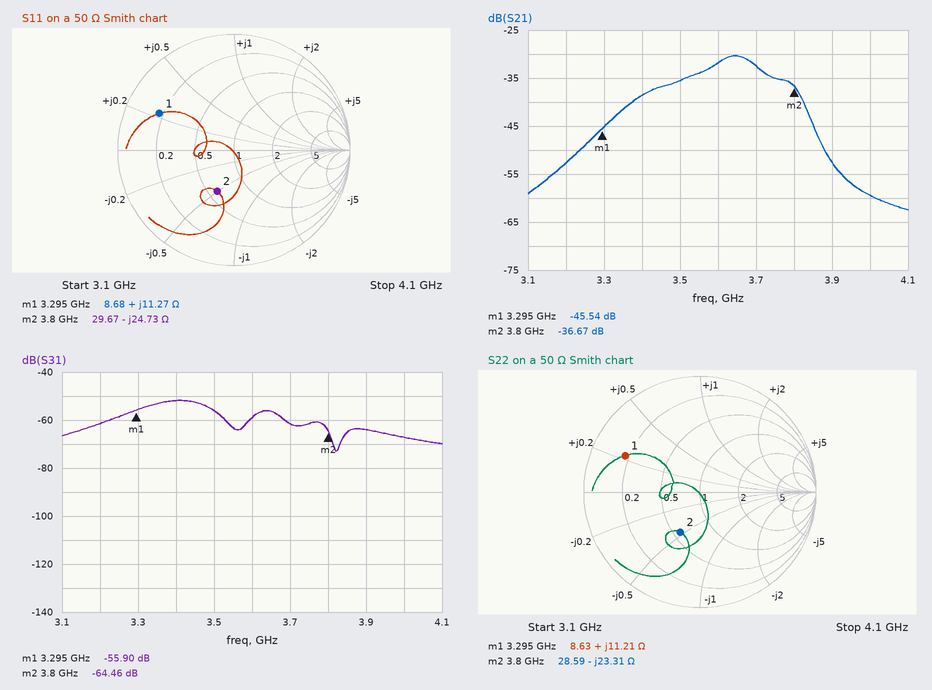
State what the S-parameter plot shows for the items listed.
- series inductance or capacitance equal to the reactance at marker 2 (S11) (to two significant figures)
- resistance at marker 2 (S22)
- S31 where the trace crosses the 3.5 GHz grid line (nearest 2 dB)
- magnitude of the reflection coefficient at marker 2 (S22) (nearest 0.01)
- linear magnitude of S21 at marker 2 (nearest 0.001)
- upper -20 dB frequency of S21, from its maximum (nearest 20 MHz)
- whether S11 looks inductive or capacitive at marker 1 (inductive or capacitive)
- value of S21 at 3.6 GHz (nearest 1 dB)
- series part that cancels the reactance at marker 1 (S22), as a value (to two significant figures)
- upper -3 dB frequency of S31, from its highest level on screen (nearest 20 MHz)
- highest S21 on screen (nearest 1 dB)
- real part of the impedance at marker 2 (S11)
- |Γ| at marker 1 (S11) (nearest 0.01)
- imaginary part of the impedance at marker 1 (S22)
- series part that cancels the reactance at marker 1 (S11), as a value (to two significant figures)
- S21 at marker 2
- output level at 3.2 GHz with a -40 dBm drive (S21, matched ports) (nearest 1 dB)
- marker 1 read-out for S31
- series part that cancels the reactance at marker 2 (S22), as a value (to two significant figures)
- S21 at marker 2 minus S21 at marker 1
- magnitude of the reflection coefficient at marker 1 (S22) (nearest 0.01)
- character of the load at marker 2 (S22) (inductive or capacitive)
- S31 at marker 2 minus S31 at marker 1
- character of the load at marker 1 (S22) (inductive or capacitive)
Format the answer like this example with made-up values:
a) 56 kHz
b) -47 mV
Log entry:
a) 1.7 pF
b) 28.59 Ω
c) -56 dB
d) 0.39
e) 0.015
f) 3.88 GHz
g) inductive
h) -32 dB
i) 4.3 pF
j) 3.48 GHz
k) -30 dB
l) 29.67 Ω
m) 0.72
n) +11.21 Ω
o) 4.3 pF
p) -36.67 dB
q) -93 dBm
r) -55.90 dB
s) 980 pH
t) 8.87 dB
u) 0.72
v) capacitive
w) -8.56 dB
x) inductive
